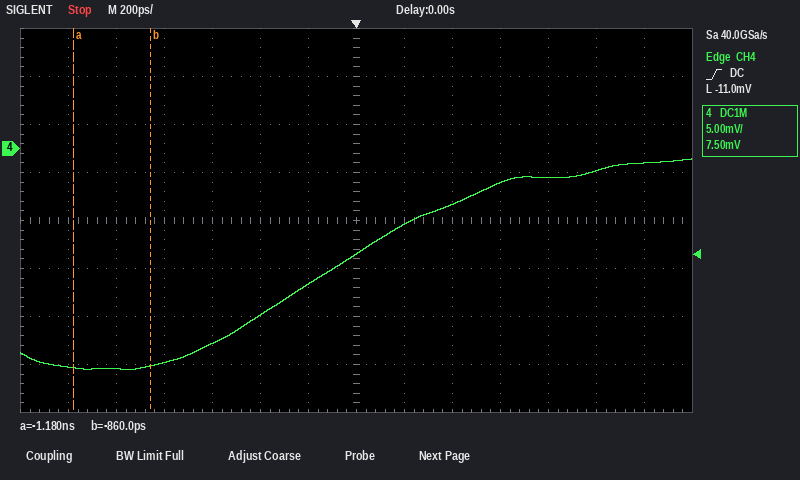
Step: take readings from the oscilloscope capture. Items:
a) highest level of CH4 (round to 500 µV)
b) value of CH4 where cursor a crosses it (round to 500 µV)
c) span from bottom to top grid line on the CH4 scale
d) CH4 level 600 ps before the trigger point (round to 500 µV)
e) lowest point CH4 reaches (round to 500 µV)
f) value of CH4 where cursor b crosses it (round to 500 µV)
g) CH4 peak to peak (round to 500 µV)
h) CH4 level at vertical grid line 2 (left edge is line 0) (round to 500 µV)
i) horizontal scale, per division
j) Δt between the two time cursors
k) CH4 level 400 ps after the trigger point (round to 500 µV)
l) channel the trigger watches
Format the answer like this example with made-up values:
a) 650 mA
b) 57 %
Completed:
a) -1.0 mV
b) -23.0 mV
c) 40 mV
d) -20.5 mV
e) -23.0 mV
f) -22.5 mV
g) 22.0 mV
h) -23.0 mV
i) 200 ps
j) 320 ps
k) -6.0 mV
l) CH4
